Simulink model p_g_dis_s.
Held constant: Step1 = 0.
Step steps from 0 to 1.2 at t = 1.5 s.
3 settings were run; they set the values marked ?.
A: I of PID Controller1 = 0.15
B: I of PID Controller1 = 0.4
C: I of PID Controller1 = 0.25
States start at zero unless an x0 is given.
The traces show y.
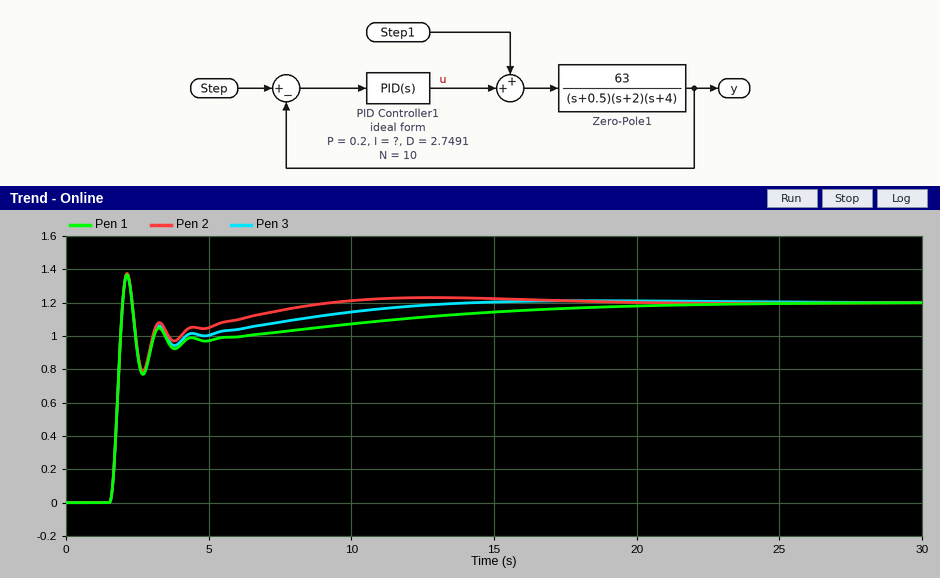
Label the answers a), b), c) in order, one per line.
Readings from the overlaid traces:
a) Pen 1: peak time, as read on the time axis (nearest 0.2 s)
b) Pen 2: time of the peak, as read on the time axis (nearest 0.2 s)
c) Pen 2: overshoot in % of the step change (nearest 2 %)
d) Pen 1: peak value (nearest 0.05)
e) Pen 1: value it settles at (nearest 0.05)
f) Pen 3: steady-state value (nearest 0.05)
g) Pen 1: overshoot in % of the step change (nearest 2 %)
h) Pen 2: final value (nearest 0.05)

a) 2.2 s
b) 2.2 s
c) 14 %
d) 1.35
e) 1.20
f) 1.20
g) 14 %
h) 1.20
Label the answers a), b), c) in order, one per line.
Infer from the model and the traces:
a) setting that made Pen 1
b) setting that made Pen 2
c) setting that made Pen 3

a) A
b) B
c) C
